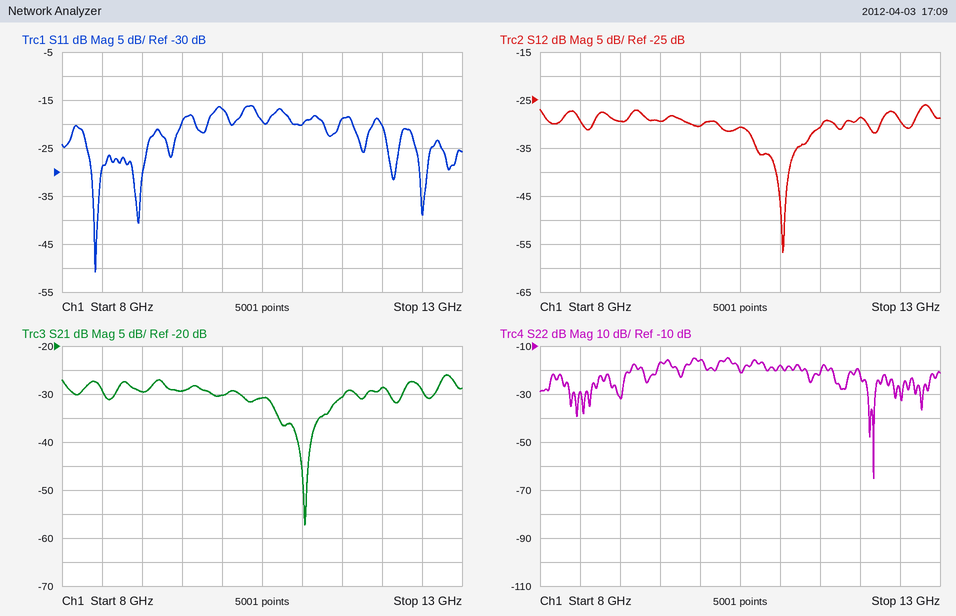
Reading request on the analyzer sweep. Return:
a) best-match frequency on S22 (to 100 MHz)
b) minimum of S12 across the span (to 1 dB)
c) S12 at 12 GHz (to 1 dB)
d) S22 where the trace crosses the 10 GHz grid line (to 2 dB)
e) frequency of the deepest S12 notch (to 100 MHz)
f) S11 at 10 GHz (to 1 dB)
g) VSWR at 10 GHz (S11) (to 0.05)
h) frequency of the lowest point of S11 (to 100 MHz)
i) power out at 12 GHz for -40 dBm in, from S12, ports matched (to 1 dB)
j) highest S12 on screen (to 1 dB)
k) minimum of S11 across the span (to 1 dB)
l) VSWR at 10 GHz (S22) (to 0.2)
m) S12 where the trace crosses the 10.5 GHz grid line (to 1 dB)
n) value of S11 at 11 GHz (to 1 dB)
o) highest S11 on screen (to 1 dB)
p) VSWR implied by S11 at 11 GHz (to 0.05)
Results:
12.2 GHz
-57 dB
-29 dB
-16 dB
11.0 GHz
-17 dB
1.35
8.4 GHz
-69 dBm
-26 dB
-51 dB
1.4
-31 dB
-20 dB
-16 dB
1.20
